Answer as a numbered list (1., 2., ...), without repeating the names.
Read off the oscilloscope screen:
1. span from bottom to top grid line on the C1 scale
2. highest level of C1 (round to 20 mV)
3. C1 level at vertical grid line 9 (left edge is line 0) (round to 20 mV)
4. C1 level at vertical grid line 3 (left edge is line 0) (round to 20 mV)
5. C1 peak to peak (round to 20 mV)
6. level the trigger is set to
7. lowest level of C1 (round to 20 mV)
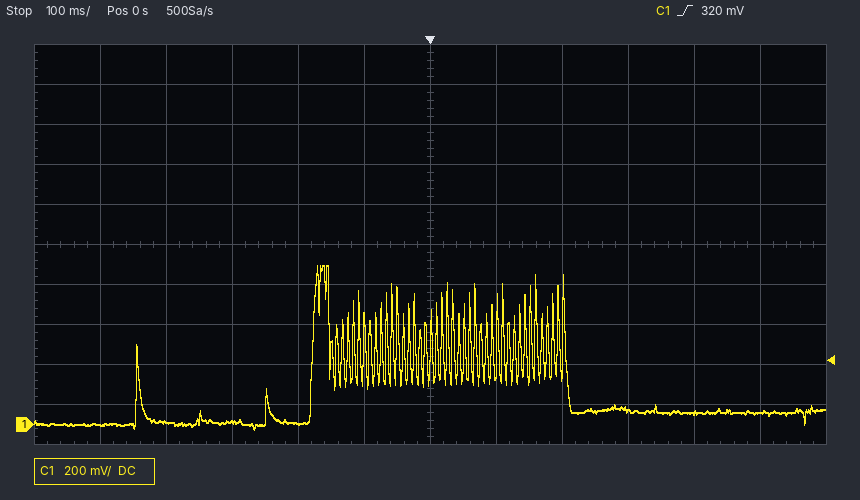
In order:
1. 2 V
2. 800 mV
3. 80 mV
4. 20 mV
5. 820 mV
6. 320 mV
7. -20 mV
